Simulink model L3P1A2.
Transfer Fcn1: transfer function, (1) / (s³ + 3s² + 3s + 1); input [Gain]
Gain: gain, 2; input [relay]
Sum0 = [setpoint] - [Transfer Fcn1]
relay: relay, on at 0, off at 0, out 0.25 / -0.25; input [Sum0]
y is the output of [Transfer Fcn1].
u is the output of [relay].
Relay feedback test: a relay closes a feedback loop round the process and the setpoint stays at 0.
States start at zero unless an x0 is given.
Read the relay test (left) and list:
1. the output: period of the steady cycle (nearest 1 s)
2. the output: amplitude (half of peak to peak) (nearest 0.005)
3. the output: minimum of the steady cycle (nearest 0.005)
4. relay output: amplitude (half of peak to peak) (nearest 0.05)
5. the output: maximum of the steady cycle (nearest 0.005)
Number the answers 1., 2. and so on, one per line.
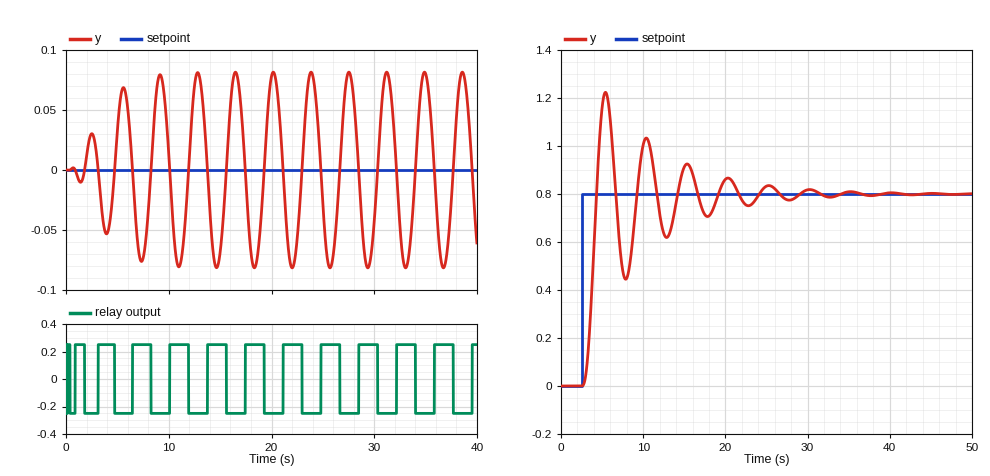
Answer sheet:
1. 4 s
2. 0.080
3. -0.080
4. 0.25
5. 0.080
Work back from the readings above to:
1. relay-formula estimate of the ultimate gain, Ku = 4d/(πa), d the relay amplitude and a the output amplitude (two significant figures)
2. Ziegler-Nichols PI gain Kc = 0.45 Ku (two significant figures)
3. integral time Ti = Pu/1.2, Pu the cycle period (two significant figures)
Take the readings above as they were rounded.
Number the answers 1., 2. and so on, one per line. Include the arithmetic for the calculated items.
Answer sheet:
1. 4 × 0.25 / (π × 0.08) = 4.0
2. 0.45 × 4 = 1.8
3. 4 / 1.2 = 3.3 s
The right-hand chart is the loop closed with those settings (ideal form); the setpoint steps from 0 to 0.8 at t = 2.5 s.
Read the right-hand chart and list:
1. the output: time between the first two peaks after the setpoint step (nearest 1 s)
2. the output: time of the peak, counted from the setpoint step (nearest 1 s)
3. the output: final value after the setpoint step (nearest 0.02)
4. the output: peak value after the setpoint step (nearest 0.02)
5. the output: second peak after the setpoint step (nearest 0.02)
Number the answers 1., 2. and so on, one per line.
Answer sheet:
1. 5 s
2. 3 s
3. 0.80
4. 1.22
5. 1.04
